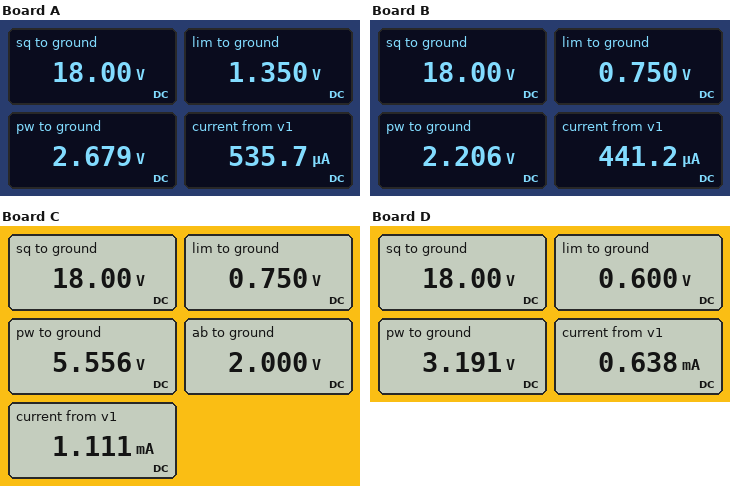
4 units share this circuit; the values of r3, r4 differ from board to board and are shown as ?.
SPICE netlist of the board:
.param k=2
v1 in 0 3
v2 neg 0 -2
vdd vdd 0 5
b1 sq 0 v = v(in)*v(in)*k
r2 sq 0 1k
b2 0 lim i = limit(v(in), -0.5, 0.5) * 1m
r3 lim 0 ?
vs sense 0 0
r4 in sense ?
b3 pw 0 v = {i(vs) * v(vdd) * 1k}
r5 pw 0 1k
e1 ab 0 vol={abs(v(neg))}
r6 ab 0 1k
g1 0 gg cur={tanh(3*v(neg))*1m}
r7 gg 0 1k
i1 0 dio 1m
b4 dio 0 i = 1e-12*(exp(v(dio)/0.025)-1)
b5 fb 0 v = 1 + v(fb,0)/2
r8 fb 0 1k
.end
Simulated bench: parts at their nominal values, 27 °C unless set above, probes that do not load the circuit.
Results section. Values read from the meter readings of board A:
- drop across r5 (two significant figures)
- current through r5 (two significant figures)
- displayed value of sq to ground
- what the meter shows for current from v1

2.7 V
2.7 mA
18.00 V
535.7 µA
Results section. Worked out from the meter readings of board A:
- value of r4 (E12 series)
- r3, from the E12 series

5.6 kΩ
2.7 kΩ
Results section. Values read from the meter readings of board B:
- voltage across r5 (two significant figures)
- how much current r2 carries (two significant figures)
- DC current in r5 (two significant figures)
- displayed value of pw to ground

2.2 V
18 mA
2.2 mA
2.206 V
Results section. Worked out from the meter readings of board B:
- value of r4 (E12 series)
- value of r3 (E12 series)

6.8 kΩ
1.5 kΩ
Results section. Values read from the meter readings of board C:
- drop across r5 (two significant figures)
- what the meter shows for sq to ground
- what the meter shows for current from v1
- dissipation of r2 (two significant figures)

5.6 V
18.00 V
1.111 mA
320 mW
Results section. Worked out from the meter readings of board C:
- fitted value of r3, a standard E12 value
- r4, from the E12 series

1.5 kΩ
2.7 kΩ
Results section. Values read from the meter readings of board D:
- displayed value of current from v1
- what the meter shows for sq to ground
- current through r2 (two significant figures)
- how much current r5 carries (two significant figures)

0.638 mA
18.00 V
18 mA
3.2 mA
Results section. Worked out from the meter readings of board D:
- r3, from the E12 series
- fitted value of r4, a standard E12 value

1.2 kΩ
4.7 kΩ
